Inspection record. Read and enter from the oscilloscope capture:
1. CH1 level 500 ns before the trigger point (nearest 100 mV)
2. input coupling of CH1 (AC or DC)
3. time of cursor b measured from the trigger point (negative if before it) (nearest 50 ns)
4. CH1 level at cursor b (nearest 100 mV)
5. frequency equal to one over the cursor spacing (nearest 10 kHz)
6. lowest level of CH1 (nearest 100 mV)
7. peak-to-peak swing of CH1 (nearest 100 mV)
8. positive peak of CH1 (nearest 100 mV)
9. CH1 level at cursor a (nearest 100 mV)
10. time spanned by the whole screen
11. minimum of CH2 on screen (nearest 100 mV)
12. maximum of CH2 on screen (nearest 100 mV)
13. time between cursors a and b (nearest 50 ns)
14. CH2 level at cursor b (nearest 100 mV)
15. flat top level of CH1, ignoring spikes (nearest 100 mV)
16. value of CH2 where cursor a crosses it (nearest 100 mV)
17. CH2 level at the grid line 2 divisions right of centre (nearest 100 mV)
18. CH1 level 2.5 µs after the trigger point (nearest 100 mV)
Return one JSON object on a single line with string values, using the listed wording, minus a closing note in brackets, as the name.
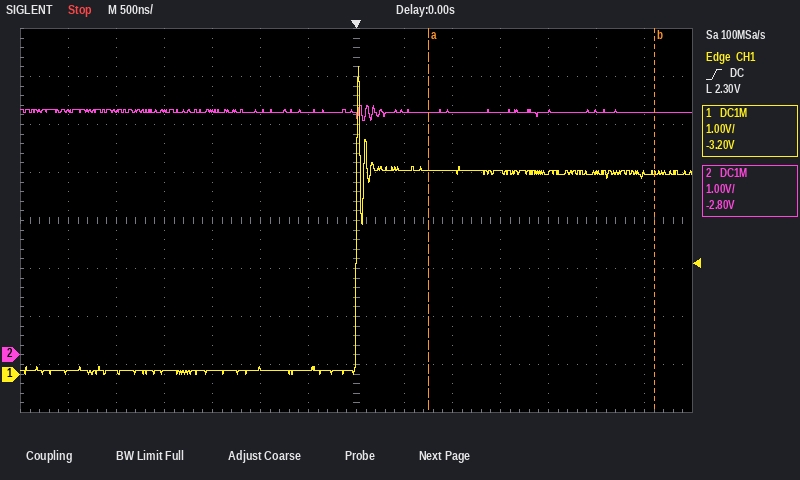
{"CH1 level 500 ns before the trigger point": "100 mV", "input coupling of CH1": "DC", "time of cursor b measured from the trigger point (negative if before it)": "+3.10 µs", "CH1 level at cursor b": "4.2 V", "frequency equal to one over the cursor spacing": "430 kHz", "lowest level of CH1": "0.0 V", "peak-to-peak swing of CH1": "6.4 V", "positive peak of CH1": "6.4 V", "CH1 level at cursor a": "4.2 V", "time spanned by the whole screen": "7 µs", "minimum of CH2 on screen": "4.9 V", "maximum of CH2 on screen": "5.2 V", "time between cursors a and b": "2.35 µs", "CH2 level at cursor b": "5.0 V", "flat top level of CH1, ignoring spikes": "4.2 V", "value of CH2 where cursor a crosses it": "5.0 V", "CH2 level at the grid line 2 divisions right of centre": "5.0 V", "CH1 level 2.5 µs after the trigger point": "4.2 V"}
